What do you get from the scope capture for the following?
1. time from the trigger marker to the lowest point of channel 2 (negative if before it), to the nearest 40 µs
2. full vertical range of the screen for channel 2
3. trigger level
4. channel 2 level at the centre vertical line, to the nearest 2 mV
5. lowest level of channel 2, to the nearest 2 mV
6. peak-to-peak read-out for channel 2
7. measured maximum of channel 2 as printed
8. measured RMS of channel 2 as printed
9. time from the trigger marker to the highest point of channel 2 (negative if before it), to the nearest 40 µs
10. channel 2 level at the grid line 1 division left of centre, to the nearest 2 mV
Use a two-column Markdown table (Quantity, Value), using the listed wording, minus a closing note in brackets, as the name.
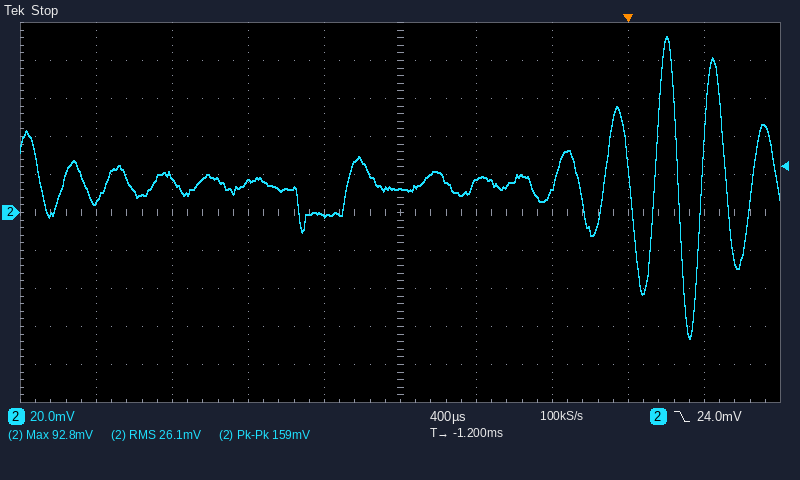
| Quantity | Value |
|---|---|
| time from the trigger marker to the lowest point of channel 2 (negative if before it), to the nearest 40 µs | +320 µs |
| full vertical range of the screen for channel 2 | 200 mV |
| trigger level | 24.0 mV |
| channel 2 level at the centre vertical line, to the nearest 2 mV | 12 mV |
| lowest level of channel 2, to the nearest 2 mV | -66 mV |
| peak-to-peak read-out for channel 2 | 159 mV |
| measured maximum of channel 2 as printed | 92.8 mV |
| measured RMS of channel 2 as printed | 26.1 mV |
| time from the trigger marker to the highest point of channel 2 (negative if before it), to the nearest 40 µs | +200 µs |
| channel 2 level at the grid line 1 division left of centre, to the nearest 2 mV | -2 mV |
